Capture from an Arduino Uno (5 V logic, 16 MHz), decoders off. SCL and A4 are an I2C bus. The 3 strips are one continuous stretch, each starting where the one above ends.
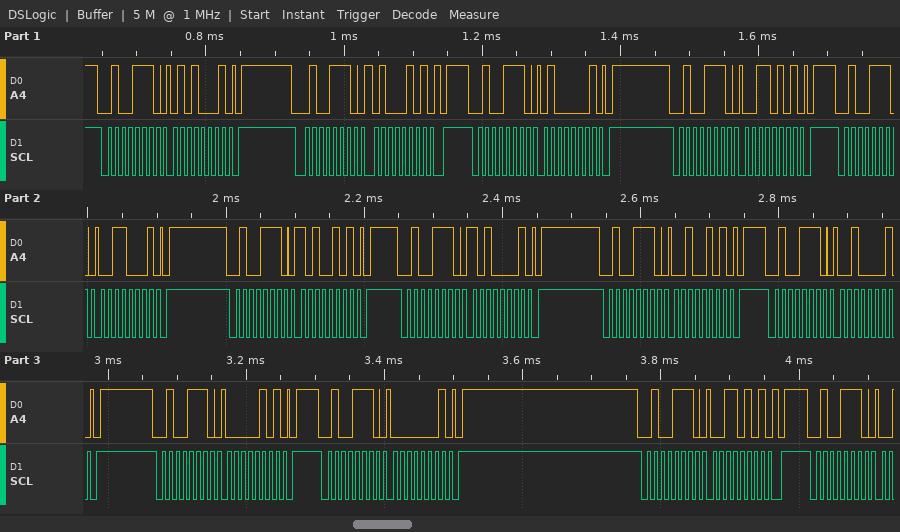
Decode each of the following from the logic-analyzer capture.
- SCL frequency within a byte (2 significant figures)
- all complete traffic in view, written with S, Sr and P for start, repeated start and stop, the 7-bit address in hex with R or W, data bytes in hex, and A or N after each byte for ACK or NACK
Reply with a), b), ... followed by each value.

a) 100 kHz
b) S 27W A 51 A P S 27W A 45 A P S 27W A 41 A P S 27W A 35 A P S 27W A 31 A P S 27W A A5 A P S 27W A A1 A P S 27W A 25 A P S 27W A 21 A P S 27W A 05 A P S 27W A 01 A P S 27W A 35 A P S 27W A
